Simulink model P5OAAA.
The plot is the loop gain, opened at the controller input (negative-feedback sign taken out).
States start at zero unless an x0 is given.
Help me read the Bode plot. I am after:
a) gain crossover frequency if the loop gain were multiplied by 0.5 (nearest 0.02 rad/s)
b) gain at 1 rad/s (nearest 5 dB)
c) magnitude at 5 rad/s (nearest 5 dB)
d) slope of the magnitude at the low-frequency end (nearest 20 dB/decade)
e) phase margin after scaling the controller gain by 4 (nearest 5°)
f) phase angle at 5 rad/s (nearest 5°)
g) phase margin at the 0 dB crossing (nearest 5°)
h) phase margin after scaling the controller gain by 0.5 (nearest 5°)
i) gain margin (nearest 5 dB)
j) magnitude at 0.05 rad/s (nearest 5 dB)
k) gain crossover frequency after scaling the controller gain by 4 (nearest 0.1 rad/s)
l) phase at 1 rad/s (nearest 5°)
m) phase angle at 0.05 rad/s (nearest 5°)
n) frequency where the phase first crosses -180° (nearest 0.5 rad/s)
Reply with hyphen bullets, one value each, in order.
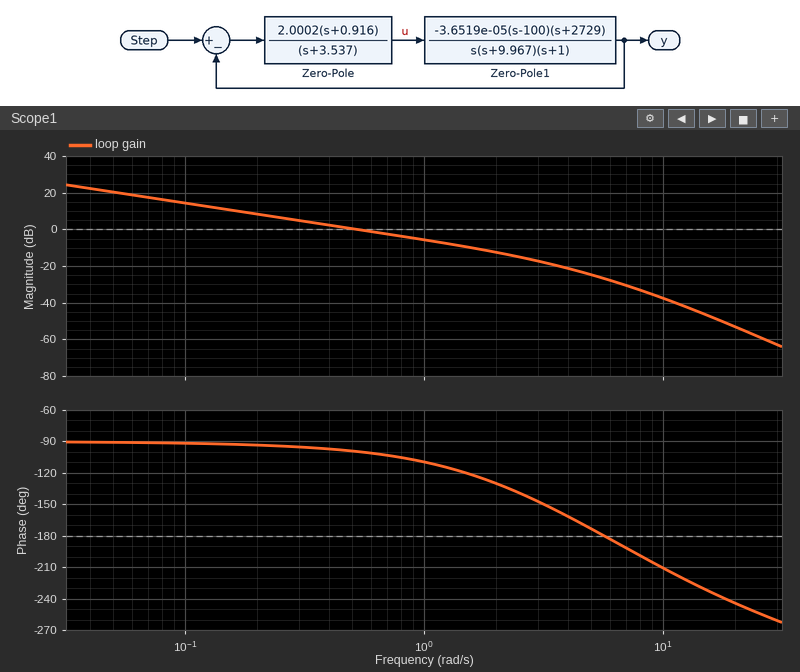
- 0.26 rad/s
- -5 dB
- -25 dB
- -20 dB/decade
- 50°
- -175°
- 80°
- 85°
- 25 dB
- 20 dB
- 1.9 rad/s
- -110°
- -90°
- 5.5 rad/s
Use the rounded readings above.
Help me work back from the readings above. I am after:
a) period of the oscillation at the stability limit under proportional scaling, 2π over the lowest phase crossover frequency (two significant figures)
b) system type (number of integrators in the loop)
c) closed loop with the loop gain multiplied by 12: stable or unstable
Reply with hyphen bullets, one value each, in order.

- 1.1 s
- 1
- stable
